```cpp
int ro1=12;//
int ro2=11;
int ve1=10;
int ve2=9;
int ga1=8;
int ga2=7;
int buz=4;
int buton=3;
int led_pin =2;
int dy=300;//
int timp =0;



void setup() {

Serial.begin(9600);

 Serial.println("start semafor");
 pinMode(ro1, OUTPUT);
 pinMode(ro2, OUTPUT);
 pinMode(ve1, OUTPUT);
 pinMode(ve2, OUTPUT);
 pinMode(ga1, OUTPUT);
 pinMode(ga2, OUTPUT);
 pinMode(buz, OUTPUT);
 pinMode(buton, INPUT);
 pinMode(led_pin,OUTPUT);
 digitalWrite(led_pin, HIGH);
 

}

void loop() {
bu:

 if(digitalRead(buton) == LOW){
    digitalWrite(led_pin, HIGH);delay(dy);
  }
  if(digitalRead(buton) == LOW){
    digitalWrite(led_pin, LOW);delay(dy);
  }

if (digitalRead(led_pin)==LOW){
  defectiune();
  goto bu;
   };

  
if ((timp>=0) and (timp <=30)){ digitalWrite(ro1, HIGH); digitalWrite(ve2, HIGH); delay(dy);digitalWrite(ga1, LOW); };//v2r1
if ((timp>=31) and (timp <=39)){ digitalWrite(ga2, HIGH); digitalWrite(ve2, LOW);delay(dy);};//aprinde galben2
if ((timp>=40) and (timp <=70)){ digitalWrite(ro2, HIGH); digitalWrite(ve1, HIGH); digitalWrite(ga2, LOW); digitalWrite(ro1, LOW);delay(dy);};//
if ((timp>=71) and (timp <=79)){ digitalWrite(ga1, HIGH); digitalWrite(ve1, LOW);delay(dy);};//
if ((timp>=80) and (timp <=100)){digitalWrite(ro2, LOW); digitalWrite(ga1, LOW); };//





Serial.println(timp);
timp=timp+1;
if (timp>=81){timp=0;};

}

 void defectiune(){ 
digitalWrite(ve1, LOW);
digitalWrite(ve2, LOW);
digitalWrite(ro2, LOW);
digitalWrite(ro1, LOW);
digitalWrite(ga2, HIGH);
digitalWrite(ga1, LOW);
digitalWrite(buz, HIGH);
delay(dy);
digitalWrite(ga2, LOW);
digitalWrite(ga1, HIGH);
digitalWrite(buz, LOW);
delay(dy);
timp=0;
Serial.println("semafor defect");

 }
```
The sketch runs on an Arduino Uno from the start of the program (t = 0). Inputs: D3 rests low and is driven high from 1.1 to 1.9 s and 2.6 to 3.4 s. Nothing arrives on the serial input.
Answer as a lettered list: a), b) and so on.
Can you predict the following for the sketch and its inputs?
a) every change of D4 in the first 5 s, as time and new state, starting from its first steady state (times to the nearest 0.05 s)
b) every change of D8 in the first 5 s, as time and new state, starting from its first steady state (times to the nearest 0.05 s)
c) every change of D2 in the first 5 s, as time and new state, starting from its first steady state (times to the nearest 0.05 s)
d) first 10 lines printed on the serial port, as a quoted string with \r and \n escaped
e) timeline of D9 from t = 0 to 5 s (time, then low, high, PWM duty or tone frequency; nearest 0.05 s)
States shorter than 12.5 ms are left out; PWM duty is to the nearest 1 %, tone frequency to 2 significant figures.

a) 0 s low; 0.6 s high; 0.9 s low; 1.2 s high; 1.5 s low; 1.8 s high; 2.1 s low; 4.2 s high; 4.5 s low
b) 0 s low; 0.9 s high; 1.2 s low; 1.5 s high; 1.8 s low; 2.1 s high; 3 s low; 4.5 s high
c) 0 s high; 0.3 s low; 2.4 s high; 3.9 s low; 4.8 s high
d) "start semafor\r\nsemafor defect\r\nsemafor defect\r\nsemafor defect\r\n0\r\n1\r\n2\r\nsemafor defect\r\nsemafor defect\r\nsemafor defect\r\n"
e) 0 s low; 2.7 s high; 4.2 s low
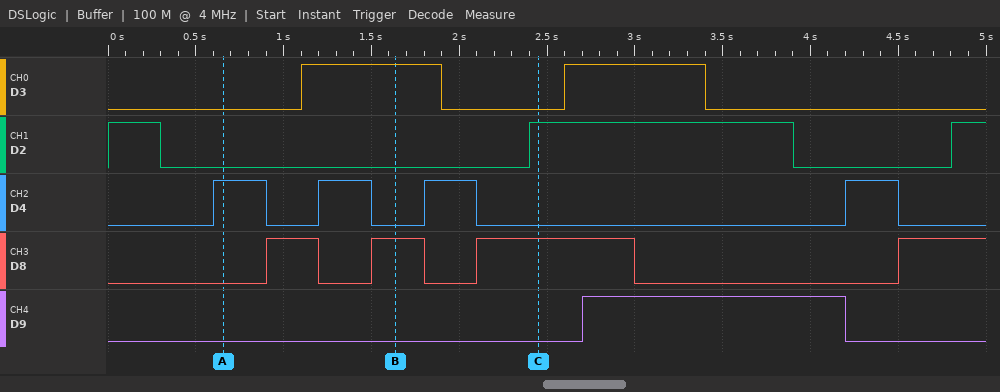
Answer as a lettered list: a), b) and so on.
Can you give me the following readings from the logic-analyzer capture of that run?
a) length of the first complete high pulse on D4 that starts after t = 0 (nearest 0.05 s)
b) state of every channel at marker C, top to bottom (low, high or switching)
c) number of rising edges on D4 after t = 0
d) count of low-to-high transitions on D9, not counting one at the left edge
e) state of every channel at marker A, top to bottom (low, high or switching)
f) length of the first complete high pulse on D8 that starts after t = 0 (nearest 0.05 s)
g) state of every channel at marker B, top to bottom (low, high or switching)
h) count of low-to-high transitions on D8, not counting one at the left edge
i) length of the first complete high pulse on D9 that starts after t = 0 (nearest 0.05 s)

a) 0.30 s
b) D3 low, D2 high, D4 low, D8 high, D9 low
c) 4
d) 1
e) D3 low, D2 low, D4 high, D8 low, D9 low
f) 0.30 s
g) D3 high, D2 low, D4 low, D8 high, D9 low
h) 4
i) 1.50 s
